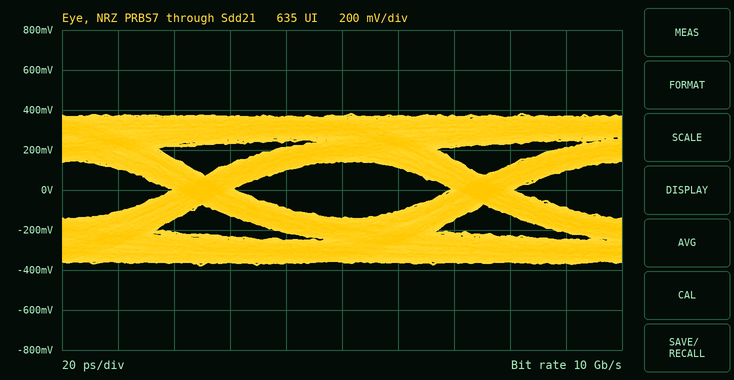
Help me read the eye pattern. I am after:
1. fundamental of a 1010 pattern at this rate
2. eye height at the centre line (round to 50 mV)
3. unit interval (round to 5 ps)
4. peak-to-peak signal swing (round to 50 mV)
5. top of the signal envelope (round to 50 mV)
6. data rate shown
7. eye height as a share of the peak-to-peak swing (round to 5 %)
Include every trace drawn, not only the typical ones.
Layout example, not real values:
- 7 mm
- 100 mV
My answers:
- 5 GHz
- 300 mV
- 100 ps
- 750 mV
- 400 mV
- 10 Gb/s
- 40 %
